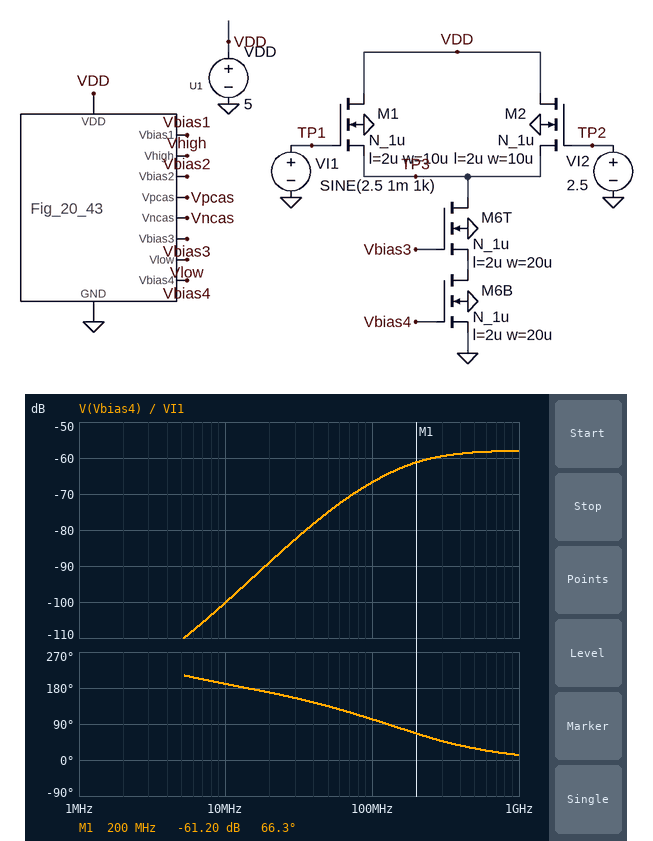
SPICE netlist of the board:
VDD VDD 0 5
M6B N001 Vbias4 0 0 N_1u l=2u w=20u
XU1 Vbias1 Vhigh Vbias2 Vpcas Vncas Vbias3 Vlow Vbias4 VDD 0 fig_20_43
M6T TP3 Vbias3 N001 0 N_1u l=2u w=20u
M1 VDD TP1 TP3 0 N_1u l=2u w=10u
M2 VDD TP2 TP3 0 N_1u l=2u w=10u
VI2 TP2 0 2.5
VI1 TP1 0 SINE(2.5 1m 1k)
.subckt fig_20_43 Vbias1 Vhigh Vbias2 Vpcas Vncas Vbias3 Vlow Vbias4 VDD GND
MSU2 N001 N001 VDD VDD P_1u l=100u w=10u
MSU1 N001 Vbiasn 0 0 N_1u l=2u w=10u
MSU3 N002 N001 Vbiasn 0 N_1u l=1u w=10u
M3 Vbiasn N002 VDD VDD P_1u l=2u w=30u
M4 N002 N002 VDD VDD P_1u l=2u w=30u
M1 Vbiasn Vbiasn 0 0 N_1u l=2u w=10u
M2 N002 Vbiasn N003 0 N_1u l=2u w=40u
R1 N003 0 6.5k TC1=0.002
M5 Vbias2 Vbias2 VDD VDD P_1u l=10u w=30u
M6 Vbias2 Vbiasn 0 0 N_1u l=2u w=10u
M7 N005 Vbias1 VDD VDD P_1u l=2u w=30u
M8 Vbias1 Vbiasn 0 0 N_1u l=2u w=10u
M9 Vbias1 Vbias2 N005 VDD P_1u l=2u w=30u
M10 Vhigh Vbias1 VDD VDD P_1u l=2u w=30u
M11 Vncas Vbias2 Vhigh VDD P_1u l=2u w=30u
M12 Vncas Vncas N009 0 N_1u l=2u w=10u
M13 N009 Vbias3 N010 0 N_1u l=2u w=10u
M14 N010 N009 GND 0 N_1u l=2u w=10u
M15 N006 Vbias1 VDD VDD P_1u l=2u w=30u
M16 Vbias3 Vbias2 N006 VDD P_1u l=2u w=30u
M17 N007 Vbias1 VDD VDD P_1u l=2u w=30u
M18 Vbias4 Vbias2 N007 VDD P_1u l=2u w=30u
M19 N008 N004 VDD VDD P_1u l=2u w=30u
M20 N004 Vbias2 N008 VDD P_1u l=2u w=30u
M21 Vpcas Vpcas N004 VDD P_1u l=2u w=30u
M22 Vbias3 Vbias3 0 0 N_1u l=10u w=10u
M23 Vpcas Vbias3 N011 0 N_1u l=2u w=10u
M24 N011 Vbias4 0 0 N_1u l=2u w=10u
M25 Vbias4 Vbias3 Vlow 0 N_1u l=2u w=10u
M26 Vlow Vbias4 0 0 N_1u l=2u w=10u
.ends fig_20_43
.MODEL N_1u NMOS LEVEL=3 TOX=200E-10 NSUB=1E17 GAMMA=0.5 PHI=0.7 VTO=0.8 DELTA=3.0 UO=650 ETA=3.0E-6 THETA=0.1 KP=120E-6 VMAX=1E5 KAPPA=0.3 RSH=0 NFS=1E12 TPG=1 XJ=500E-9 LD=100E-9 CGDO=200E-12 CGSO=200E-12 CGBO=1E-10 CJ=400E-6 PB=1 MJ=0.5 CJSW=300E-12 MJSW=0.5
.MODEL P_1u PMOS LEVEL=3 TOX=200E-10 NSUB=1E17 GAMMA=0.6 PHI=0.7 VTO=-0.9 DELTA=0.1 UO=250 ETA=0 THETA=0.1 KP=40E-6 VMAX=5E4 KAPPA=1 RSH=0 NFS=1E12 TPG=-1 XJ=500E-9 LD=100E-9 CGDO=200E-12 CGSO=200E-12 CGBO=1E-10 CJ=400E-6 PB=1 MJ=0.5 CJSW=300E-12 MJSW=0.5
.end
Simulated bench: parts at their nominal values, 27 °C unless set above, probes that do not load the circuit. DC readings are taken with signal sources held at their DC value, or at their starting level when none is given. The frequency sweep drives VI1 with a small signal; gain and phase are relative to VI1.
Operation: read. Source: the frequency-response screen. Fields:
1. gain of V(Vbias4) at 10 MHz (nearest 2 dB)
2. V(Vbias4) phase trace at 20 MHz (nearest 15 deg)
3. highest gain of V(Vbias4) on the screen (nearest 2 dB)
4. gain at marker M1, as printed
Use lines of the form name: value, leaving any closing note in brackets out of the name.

gain of V(Vbias4) at 10 MHz: -100 dB
V(Vbias4) phase trace at 20 MHz: 165 deg
highest gain of V(Vbias4) on the screen: -58 dB
gain at marker M1, as printed: -61.20 dB
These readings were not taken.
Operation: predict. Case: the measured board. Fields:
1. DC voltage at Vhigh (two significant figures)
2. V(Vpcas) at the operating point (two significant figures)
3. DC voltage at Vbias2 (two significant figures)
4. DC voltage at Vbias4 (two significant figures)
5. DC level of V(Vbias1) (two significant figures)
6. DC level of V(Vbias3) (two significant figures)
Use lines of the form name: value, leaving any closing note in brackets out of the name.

DC voltage at Vhigh: 4.7 V
V(Vpcas) at the operating point: 2.4 V
DC voltage at Vbias2: 3.4 V
DC voltage at Vbias4: 1.1 V
DC level of V(Vbias1): 3.8 V
DC level of V(Vbias3): 1.5 V
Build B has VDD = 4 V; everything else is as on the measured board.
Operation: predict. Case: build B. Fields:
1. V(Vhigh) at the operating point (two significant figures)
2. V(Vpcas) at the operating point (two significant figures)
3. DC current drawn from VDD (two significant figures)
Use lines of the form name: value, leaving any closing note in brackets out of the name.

V(Vhigh) at the operating point: 3.7 V
V(Vpcas) at the operating point: 1.4 V
DC current drawn from VDD: 220 µA
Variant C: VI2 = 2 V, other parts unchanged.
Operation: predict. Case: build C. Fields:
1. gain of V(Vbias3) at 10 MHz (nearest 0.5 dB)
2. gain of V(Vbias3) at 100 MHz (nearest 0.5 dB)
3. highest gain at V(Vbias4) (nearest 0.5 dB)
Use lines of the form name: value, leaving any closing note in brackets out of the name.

gain of V(Vbias3) at 10 MHz: -49.0 dB
gain of V(Vbias3) at 100 MHz: -34.5 dB
highest gain at V(Vbias4): -53.0 dB
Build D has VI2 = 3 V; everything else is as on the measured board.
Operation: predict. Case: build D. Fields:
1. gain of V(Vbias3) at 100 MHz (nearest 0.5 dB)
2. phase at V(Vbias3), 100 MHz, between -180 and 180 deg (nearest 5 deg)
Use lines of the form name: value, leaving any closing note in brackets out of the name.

gain of V(Vbias3) at 100 MHz: -61.5 dB
phase at V(Vbias3), 100 MHz, between -180 and 180 deg: 105 deg
